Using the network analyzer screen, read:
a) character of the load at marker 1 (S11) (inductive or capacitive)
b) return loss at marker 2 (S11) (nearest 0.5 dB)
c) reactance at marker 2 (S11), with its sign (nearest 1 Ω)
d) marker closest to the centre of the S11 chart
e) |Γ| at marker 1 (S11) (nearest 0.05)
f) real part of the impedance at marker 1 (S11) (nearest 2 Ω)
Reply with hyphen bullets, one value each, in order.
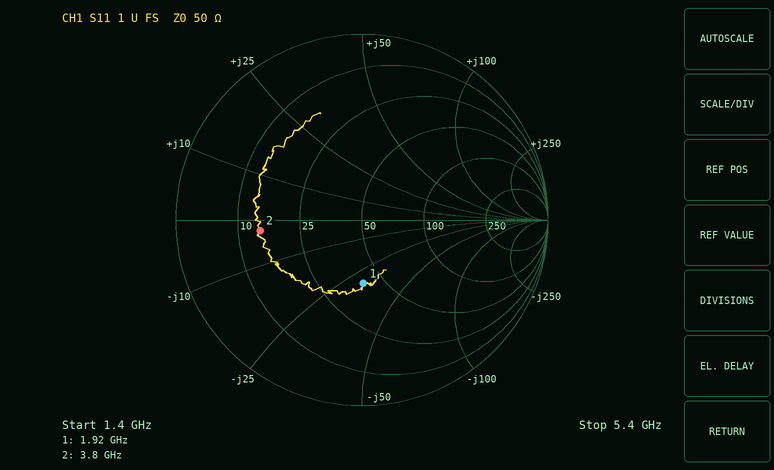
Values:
- capacitive
- 5.0 dB
- -2 Ω
- marker 1
- 0.35
- 40 Ω
